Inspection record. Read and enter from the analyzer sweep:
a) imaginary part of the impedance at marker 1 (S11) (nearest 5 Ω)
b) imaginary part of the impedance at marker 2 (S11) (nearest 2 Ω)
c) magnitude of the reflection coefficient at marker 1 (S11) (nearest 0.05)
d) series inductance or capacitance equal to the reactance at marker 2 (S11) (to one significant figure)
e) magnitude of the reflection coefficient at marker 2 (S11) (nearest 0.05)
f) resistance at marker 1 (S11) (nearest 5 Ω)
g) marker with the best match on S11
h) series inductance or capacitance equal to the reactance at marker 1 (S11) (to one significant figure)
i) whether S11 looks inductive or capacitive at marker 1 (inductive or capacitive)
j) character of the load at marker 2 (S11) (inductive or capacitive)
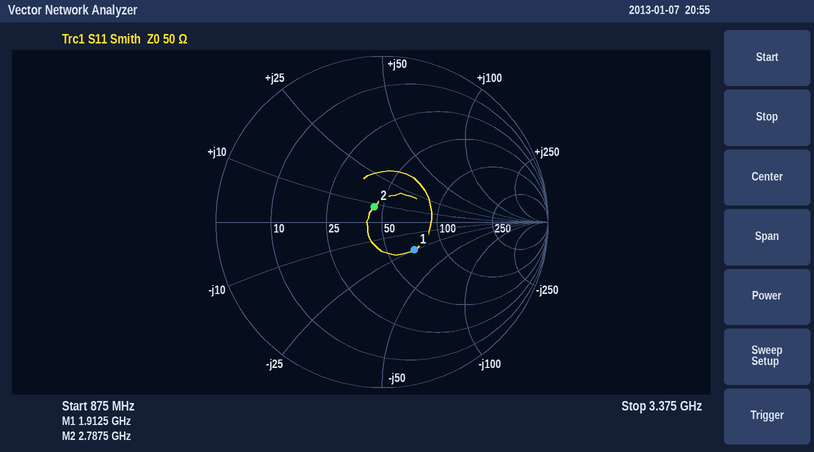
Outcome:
-25 Ω
+8 Ω
0.25
500 pH
0.10
70 Ω
marker 2
3 pF
capacitive
inductive
